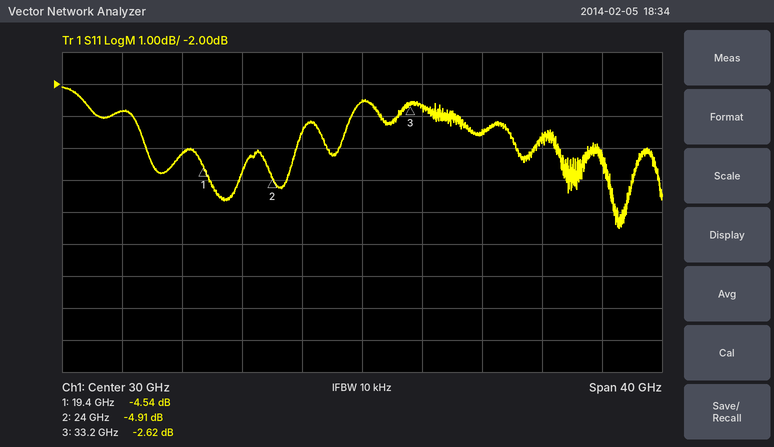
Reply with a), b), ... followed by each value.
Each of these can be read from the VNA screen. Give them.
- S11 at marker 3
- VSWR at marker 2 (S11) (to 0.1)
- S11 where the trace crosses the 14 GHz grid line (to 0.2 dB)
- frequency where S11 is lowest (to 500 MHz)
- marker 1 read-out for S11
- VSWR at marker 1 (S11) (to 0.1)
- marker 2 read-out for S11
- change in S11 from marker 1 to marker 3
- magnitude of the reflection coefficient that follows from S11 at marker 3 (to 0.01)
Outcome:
a) -2.62 dB
b) 3.6
c) -2.8 dB
d) 47.0 GHz
e) -4.54 dB
f) 3.9
g) -4.91 dB
h) 1.92 dB
i) 0.74
